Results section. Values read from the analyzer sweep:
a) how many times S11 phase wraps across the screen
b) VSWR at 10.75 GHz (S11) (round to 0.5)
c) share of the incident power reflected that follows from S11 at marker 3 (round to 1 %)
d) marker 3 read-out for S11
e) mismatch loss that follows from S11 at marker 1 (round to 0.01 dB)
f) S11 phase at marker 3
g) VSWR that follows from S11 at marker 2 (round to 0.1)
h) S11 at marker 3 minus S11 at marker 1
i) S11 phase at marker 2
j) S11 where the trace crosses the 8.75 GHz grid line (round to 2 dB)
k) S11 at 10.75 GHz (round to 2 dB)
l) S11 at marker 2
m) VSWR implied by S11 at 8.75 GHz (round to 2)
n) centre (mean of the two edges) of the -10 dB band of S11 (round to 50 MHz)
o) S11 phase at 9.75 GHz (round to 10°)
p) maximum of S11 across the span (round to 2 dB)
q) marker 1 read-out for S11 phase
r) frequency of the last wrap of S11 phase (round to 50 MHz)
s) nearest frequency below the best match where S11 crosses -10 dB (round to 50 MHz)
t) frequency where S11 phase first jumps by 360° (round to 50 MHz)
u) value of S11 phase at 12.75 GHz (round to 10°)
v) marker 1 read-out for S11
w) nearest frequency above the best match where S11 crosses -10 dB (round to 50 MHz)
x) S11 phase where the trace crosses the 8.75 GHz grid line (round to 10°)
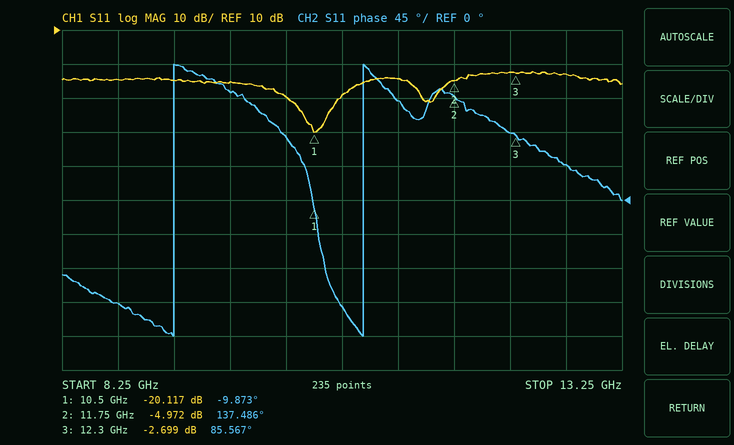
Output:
2
2.0
54 %
-2.699 dB
0.04 dB
85.567°
3.6
17.418 dB
137.486°
-4 dB
-10 dB
-4.972 dB
4
10.50 GHz
140°
-2 dB
-9.873°
10.95 GHz
10.25 GHz
9.25 GHz
50°
-20.117 dB
10.75 GHz
-140°
